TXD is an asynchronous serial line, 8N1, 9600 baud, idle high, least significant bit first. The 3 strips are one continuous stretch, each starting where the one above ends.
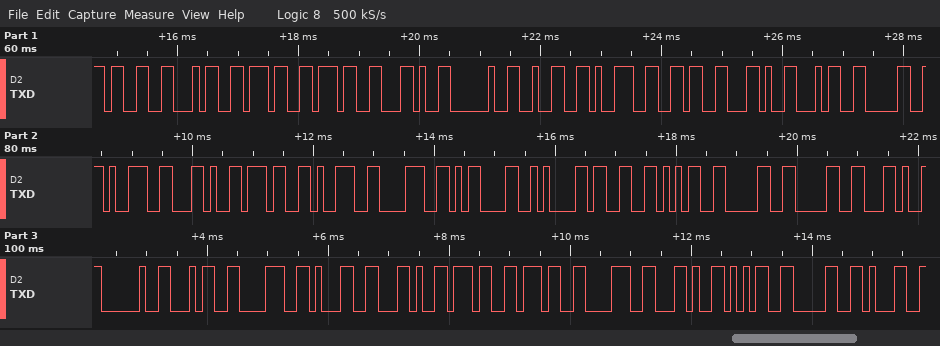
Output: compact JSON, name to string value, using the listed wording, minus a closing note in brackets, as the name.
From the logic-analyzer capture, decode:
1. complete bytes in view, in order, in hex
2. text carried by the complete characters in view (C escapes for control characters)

{"complete bytes in view, in order, in hex": "33 34 37 37 2C 20 32 39 36 2C 34 30 39 2C 37 39 38 0D 0A 33 35 30 30 2C 20 34 38 31 2C 37 37 38 2C 35 30 31", "text carried by the complete characters in view": "\"3477, 296,409,798\\r\\n3500, 481,778,501\""}
